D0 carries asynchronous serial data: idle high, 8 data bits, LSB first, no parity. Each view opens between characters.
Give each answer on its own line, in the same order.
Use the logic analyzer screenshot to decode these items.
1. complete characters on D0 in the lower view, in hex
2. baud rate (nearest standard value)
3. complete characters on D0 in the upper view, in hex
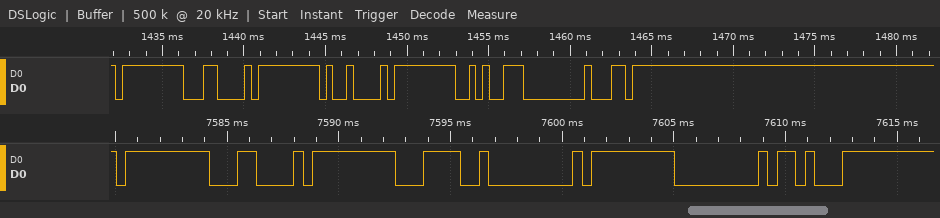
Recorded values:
FF, 0C, FF, 3C, 00, FF, 00, 8B
2400 baud
FF, 0C, FF, 09, FF, CA, 00, EC
